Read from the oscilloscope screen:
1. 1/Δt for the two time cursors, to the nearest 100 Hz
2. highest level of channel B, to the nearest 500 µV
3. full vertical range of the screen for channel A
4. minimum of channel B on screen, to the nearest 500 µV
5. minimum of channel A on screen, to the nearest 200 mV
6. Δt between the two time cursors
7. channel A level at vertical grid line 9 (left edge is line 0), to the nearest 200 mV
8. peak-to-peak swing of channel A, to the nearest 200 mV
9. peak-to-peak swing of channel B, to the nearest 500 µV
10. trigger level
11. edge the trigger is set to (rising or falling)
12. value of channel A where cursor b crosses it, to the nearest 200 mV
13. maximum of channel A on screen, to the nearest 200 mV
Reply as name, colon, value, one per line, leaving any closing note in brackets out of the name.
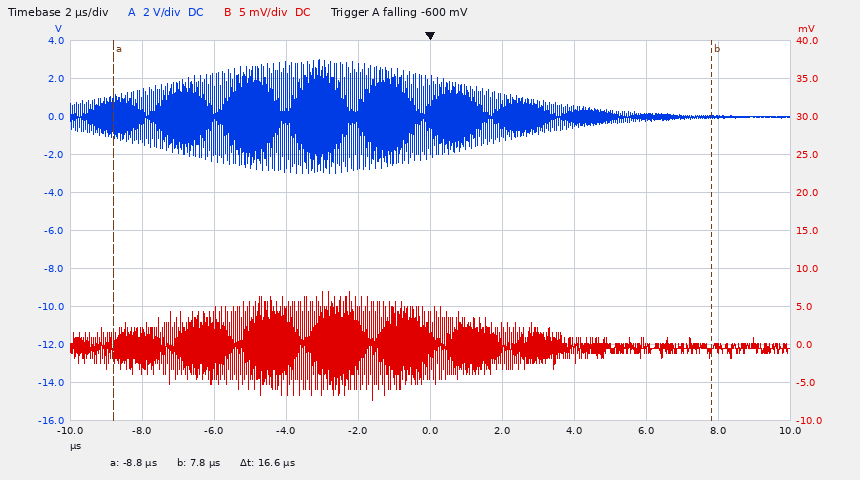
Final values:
1/Δt for the two time cursors, to the nearest 100 Hz: 60.2 kHz
highest level of channel B, to the nearest 500 µV: 7.0 mV
full vertical range of the screen for channel A: 20 V
minimum of channel B on screen, to the nearest 500 µV: -7.5 mV
minimum of channel A on screen, to the nearest 200 mV: -3.0 V
Δt between the two time cursors: 16.6 µs
channel A level at vertical grid line 9 (left edge is line 0), to the nearest 200 mV: 0.0 V
peak-to-peak swing of channel A, to the nearest 200 mV: 6.0 V
peak-to-peak swing of channel B, to the nearest 500 µV: 14.5 mV
trigger level: -600 mV
edge the trigger is set to: falling
value of channel A where cursor b crosses it, to the nearest 200 mV: 0.0 V
maximum of channel A on screen, to the nearest 200 mV: 3.0 V
